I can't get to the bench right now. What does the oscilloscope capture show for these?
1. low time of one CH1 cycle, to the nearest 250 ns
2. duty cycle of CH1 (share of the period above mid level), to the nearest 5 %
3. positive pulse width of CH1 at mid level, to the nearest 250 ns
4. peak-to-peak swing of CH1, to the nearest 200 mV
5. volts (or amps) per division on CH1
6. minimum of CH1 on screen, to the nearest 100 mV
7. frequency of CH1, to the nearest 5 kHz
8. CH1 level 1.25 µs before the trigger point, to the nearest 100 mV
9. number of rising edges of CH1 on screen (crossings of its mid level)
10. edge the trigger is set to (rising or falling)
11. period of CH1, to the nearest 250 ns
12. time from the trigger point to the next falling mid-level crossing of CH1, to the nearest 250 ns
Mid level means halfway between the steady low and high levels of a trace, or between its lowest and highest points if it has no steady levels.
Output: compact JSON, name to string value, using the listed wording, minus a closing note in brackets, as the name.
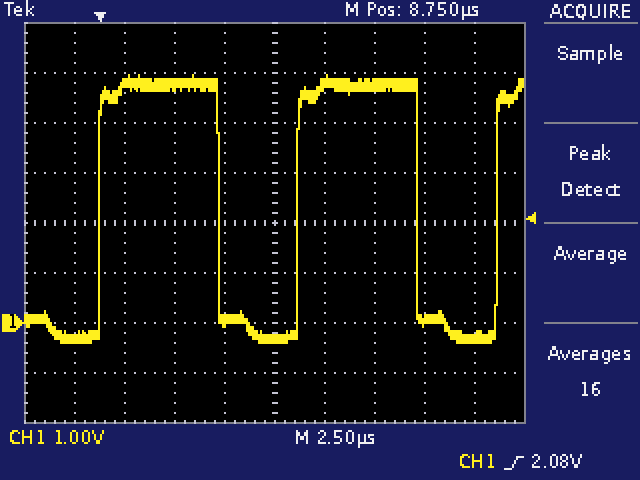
{"low time of one CH1 cycle, to the nearest 250 ns": "4.00 µs", "duty cycle of CH1 (share of the period above mid level), to the nearest 5 %": "60 %", "positive pulse width of CH1 at mid level, to the nearest 250 ns": "6.00 µs", "peak-to-peak swing of CH1, to the nearest 200 mV": "5.4 V", "volts (or amps) per division on CH1": "1 V", "minimum of CH1 on screen, to the nearest 100 mV": "-400 mV", "frequency of CH1, to the nearest 5 kHz": "100 kHz", "CH1 level 1.25 µs before the trigger point, to the nearest 100 mV": "-300 mV", "number of rising edges of CH1 on screen": "3", "edge the trigger is set to": "rising", "period of CH1, to the nearest 250 ns": "10.00 µs", "time from the trigger point to the next falling mid-level crossing of CH1, to the nearest 250 ns": "6.00 µs"}
